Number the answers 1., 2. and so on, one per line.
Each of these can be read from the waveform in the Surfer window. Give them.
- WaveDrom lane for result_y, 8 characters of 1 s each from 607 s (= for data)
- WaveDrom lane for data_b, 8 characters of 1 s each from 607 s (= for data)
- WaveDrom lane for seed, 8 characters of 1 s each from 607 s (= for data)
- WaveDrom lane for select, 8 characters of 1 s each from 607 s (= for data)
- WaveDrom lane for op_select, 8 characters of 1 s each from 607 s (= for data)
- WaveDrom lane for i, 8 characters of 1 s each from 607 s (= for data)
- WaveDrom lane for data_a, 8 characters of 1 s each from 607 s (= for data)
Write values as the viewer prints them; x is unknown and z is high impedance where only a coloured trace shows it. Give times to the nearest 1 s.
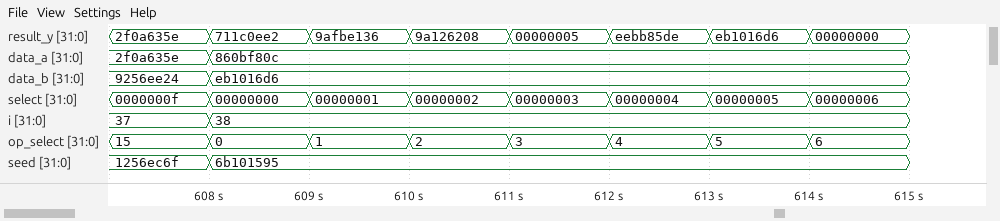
1. {name: 'result_y', wave: '========', data: '2f0a635e 711c0ee2 9afbe136 9a126208 00000005 eebb85de eb1016d6 00000000'}
2. {name: 'data_b', wave: '==......', data: '9256ee24 eb1016d6'}
3. {name: 'seed', wave: '==......', data: '1256ec6f 6b101595'}
4. {name: 'select', wave: '========', data: '0000000f 00000000 00000001 00000002 00000003 00000004 00000005 00000006'}
5. {name: 'op_select', wave: '========', data: '15 0 1 2 3 4 5 6'}
6. {name: 'i', wave: '==......', data: '37 38'}
7. {name: 'data_a', wave: '==......', data: '2f0a635e 860bf80c'}
